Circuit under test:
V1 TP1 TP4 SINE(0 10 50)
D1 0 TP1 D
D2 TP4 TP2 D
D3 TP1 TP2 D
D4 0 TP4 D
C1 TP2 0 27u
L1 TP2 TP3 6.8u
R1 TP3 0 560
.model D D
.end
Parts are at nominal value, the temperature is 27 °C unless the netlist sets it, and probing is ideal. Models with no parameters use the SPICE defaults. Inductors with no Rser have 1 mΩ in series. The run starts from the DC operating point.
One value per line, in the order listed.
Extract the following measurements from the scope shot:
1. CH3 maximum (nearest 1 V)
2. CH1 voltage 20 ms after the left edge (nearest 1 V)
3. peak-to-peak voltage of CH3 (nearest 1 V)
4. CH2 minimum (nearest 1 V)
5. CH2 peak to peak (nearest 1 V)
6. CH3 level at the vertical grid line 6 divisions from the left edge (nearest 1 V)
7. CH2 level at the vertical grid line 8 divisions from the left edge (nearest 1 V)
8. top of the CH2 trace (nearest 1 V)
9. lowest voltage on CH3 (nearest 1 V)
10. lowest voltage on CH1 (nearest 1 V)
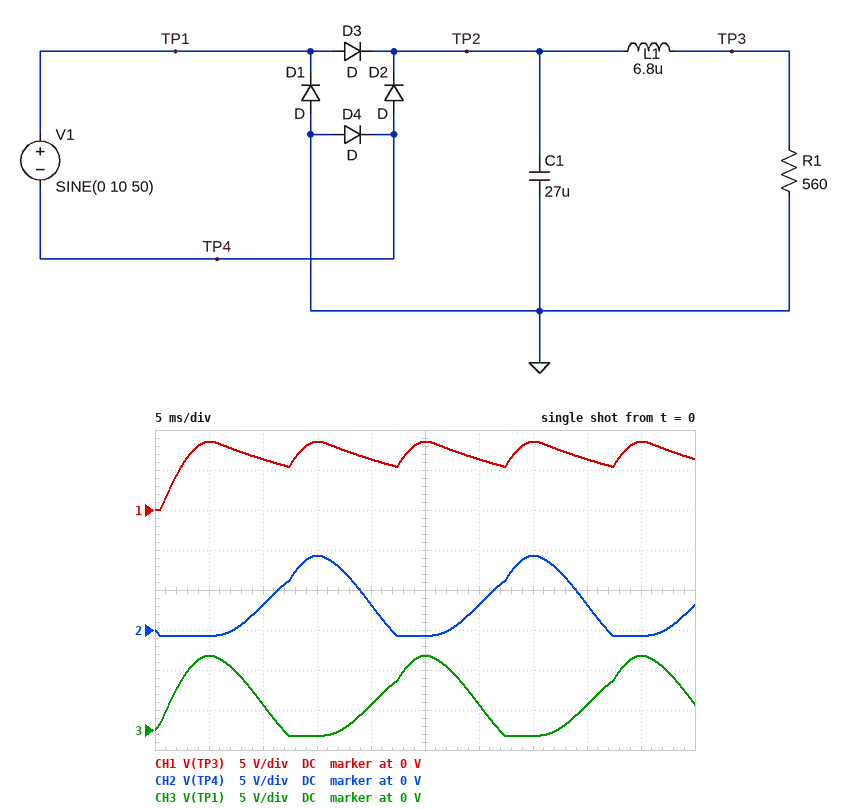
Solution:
9 V
6 V
10 V
-1 V
10 V
3 V
3 V
9 V
-1 V
0 V
